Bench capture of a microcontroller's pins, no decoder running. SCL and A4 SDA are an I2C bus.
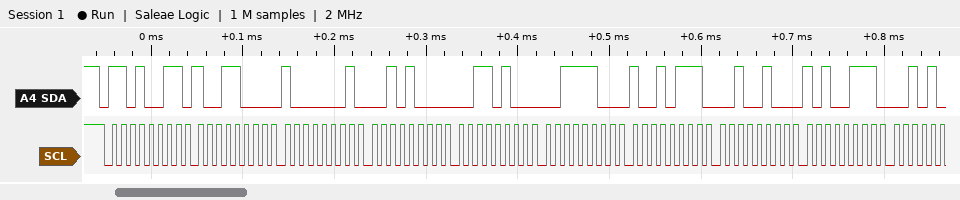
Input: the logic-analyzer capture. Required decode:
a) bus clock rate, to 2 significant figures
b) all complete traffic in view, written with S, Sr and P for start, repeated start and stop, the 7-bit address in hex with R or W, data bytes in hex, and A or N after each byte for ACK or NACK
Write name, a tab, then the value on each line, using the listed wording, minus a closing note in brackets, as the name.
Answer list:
bus clock rate, to 2 significant figures	100 kHz
all complete traffic in view, written with S, Sr and P for start, repeated start and stop, the 7-bit address in hex with R or W, data bytes in hex, and A or N after each byte for ACK or NACK	S 69R A 98 A 81 A 28 A 34 A 3C A 97 A 24 A A7 A
